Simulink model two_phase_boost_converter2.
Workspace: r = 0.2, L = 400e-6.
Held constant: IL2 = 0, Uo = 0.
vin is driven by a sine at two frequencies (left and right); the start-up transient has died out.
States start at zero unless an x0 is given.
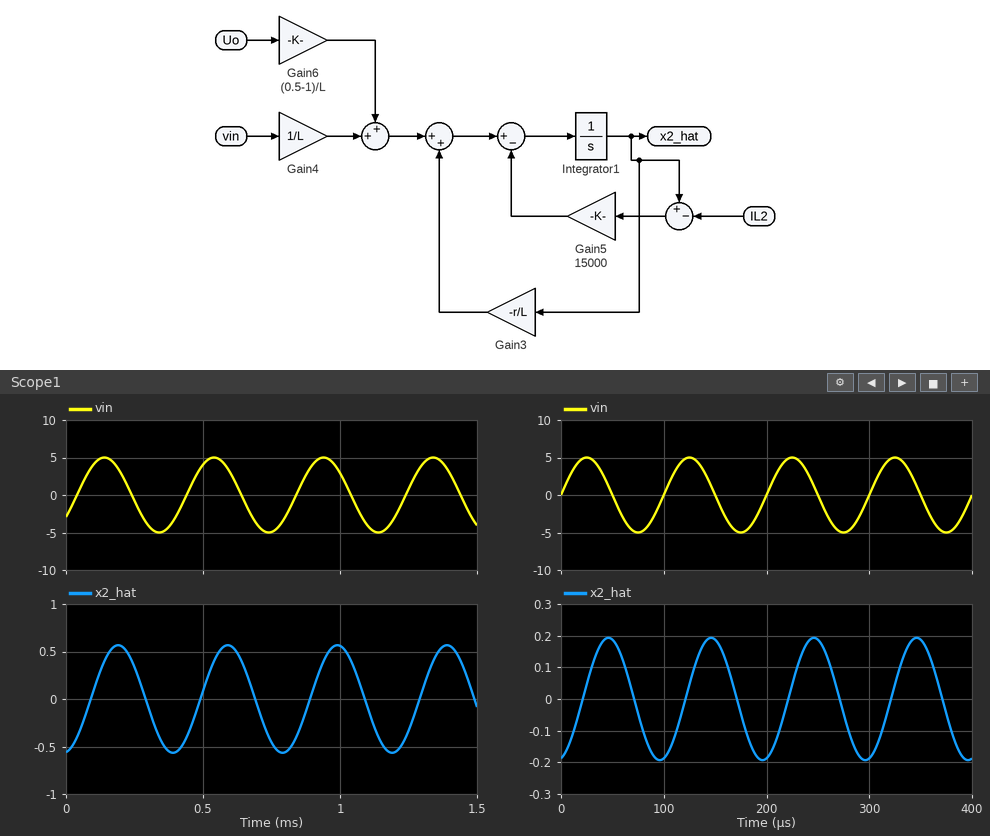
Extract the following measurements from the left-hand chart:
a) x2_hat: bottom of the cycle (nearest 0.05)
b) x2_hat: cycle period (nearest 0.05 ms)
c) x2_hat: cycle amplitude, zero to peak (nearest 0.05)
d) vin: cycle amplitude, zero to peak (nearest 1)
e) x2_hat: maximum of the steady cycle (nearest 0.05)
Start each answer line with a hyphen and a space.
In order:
- -0.55
- 0.40 ms
- 0.55
- 5
- 0.55
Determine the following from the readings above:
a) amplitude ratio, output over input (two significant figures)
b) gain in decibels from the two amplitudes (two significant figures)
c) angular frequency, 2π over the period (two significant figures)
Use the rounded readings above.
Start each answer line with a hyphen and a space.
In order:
- 0.11
- -19 dB
- 16 rad/ms
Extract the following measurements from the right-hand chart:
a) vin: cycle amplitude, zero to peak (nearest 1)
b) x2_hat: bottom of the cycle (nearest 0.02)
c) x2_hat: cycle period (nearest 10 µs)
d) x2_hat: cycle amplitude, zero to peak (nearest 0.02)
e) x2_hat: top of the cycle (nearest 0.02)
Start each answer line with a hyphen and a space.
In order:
- 5
- -0.20
- 100 µs
- 0.20
- 0.20
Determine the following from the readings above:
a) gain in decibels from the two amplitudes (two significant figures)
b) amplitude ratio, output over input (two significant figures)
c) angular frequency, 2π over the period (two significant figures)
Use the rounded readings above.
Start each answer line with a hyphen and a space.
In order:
- -28 dB
- 0.040
- 0.063 rad/µs
